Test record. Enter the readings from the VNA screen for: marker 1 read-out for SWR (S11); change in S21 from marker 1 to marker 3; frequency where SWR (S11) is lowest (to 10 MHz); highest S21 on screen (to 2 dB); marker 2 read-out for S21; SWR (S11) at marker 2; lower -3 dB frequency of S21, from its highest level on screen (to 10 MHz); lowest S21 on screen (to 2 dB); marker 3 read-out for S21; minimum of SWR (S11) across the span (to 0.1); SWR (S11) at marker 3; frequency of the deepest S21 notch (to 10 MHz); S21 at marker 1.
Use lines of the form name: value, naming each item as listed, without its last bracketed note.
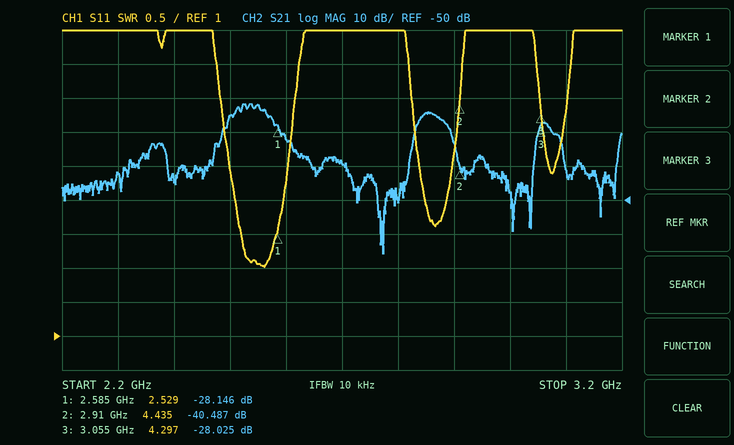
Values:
marker 1 read-out for SWR: 2.529
change in S21 from marker 1 to marker 3: 0.121 dB
frequency where SWR (S11) is lowest: 2.56 GHz
highest S21 on screen: -22 dB
marker 2 read-out for S21: -40.487 dB
SWR (S11) at marker 2: 4.435
lower -3 dB frequency of S21, from its highest level on screen: 2.51 GHz
lowest S21 on screen: -66 dB
marker 3 read-out for S21: -28.025 dB
minimum of SWR (S11) across the span: 2.0
SWR (S11) at marker 3: 4.297
frequency of the deepest S21 notch: 2.77 GHz
S21 at marker 1: -28.146 dB
